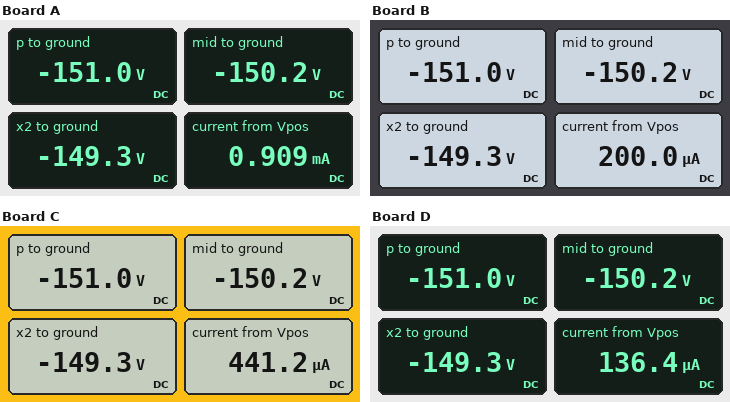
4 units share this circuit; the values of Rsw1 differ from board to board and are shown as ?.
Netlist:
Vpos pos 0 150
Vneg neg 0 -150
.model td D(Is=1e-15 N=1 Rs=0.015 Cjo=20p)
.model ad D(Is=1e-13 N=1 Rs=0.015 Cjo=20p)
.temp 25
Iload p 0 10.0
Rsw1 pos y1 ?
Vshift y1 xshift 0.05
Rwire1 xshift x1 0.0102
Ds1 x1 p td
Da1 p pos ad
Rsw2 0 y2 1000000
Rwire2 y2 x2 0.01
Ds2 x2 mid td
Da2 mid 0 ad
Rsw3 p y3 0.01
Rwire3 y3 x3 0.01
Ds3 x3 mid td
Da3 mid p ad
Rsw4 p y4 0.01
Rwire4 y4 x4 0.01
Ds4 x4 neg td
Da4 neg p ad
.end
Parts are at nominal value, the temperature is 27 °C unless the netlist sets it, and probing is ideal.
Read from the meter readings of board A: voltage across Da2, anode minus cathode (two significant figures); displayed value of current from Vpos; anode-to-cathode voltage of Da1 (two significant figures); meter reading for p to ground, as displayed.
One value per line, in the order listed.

-150 V
0.909 mA
-300 V
-151.0 V
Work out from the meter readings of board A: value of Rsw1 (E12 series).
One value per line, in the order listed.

330 kΩ
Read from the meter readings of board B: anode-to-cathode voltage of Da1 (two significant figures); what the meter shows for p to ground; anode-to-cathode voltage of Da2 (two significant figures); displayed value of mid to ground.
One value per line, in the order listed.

-300 V
-151.0 V
-150 V
-150.2 V
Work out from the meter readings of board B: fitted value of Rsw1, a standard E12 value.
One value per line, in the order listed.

1.5 MΩ
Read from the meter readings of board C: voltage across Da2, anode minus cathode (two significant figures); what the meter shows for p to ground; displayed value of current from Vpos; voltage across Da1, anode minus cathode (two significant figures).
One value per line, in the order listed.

-150 V
-151.0 V
441.2 µA
-300 V
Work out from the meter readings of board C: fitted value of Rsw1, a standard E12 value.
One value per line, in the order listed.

680 kΩ
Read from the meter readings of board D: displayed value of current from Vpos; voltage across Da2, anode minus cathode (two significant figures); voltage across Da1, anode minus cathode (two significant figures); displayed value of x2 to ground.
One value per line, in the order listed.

136.4 µA
-150 V
-300 V
-149.3 V
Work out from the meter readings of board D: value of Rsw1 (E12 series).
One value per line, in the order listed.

2.2 MΩ
